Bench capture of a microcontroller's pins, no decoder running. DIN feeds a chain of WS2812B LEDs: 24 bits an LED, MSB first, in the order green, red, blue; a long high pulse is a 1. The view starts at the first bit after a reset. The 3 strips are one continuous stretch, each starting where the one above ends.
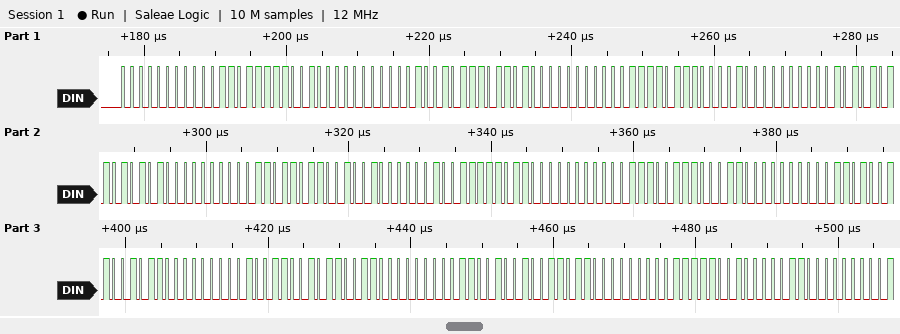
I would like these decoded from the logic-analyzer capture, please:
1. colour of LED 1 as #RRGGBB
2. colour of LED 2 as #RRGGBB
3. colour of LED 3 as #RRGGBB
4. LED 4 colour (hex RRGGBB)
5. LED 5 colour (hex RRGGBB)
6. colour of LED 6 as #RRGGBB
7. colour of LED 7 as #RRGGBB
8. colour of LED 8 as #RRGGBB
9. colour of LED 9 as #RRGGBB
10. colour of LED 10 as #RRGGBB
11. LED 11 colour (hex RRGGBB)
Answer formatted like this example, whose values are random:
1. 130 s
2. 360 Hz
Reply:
1. #1B00E4
2. #4B00B4
3. #7B0084
4. #AB0054
5. #DB0024
6. #F60900
7. #C63900
8. #966900
9. #669900
10. #36C900
11. #06F900
